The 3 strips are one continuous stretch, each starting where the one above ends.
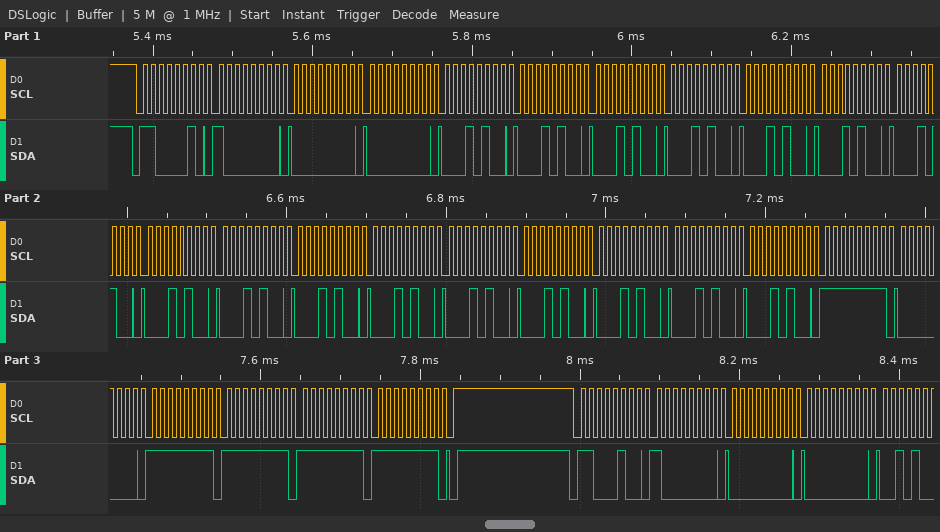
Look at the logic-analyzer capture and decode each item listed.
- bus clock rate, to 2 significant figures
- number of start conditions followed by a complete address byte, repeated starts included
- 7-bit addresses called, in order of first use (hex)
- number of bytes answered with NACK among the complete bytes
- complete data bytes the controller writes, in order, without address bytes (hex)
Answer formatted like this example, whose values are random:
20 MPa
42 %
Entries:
100 kHz
2
0x61 0x62
0
80 00 00 14 14 14 14 14 14 14 14 14 14 14 14 14 14 14 14 FF 00 FF FF FF FF 80 00 00
